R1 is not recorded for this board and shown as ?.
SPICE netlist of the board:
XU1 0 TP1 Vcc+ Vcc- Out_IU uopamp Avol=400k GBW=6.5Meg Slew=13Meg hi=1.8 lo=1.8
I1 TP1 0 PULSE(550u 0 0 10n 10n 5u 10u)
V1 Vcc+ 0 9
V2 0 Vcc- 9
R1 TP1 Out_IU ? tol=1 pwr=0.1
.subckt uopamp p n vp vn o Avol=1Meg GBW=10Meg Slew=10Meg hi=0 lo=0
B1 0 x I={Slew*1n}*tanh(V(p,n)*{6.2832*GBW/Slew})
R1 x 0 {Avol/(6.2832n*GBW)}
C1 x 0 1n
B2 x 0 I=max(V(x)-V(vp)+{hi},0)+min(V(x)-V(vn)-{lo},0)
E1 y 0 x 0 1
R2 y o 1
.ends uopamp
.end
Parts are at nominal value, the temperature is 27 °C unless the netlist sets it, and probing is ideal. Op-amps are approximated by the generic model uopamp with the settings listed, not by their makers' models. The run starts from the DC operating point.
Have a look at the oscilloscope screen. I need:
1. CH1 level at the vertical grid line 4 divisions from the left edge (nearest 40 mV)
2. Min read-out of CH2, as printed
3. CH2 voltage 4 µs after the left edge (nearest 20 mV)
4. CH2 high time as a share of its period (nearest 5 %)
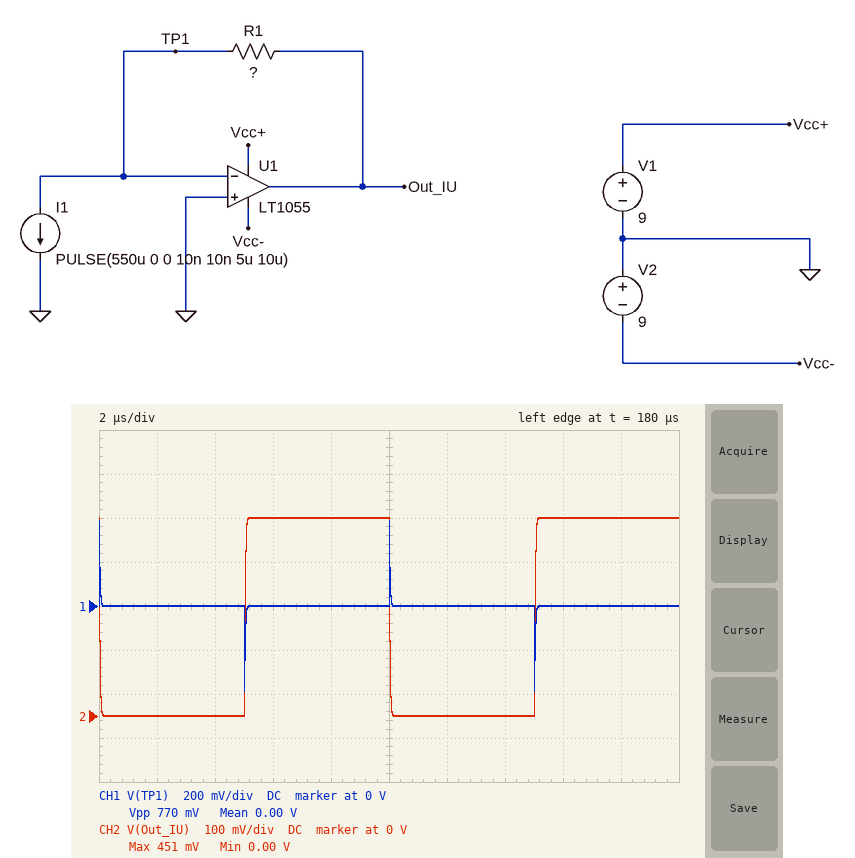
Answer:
0 V
0.00 V
0 V
50 %
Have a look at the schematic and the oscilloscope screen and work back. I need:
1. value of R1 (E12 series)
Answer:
820 Ω
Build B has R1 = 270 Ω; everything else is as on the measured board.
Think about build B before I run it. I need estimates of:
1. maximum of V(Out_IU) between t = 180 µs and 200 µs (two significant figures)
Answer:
150 mV
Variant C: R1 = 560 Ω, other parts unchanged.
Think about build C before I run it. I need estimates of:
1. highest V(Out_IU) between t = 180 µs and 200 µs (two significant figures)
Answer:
310 mV
